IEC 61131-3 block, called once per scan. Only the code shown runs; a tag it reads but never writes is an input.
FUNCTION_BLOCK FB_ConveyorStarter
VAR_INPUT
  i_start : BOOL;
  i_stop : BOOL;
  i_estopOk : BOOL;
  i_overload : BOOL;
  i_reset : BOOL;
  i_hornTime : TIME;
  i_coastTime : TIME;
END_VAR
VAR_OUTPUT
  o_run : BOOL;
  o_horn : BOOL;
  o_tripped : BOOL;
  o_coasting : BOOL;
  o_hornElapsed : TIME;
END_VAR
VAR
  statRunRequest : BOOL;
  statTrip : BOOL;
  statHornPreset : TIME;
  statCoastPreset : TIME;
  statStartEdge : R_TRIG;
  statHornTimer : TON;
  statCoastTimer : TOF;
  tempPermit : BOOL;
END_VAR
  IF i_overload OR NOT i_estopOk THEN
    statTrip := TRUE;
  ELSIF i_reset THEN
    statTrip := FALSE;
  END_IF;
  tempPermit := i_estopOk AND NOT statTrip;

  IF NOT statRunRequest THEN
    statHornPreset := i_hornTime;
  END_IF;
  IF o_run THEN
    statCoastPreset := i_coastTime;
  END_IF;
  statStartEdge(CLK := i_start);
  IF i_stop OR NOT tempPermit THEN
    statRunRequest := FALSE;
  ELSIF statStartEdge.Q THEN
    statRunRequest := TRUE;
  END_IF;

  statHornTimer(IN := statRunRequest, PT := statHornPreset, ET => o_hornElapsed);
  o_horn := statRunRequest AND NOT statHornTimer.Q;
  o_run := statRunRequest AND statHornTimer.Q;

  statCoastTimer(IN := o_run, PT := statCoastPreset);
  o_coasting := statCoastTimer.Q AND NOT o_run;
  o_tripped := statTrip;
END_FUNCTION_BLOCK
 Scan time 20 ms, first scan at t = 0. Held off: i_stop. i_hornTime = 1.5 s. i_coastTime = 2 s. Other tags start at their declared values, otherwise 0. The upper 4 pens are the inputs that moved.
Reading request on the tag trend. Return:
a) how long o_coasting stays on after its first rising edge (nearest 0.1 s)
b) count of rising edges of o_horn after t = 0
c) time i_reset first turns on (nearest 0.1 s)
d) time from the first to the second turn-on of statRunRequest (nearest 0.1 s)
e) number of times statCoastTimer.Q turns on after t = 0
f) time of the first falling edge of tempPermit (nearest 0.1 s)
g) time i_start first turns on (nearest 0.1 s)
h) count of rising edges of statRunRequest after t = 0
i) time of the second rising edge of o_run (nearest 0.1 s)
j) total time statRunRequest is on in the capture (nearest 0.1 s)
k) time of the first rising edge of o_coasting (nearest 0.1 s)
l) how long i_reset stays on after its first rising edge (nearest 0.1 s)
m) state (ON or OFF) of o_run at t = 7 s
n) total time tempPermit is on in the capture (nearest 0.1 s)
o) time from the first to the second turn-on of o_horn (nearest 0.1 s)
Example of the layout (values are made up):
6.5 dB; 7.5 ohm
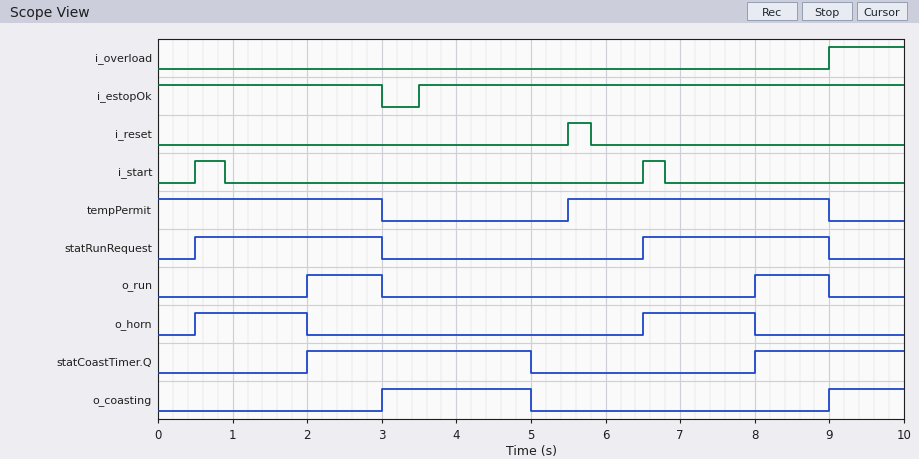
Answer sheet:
2.0 s; 2; 5.5 s; 6.0 s; 2; 3.0 s; 0.5 s; 2; 8.0 s; 5.0 s; 3.0 s; 0.3 s; OFF; 6.5 s; 6.0 s
